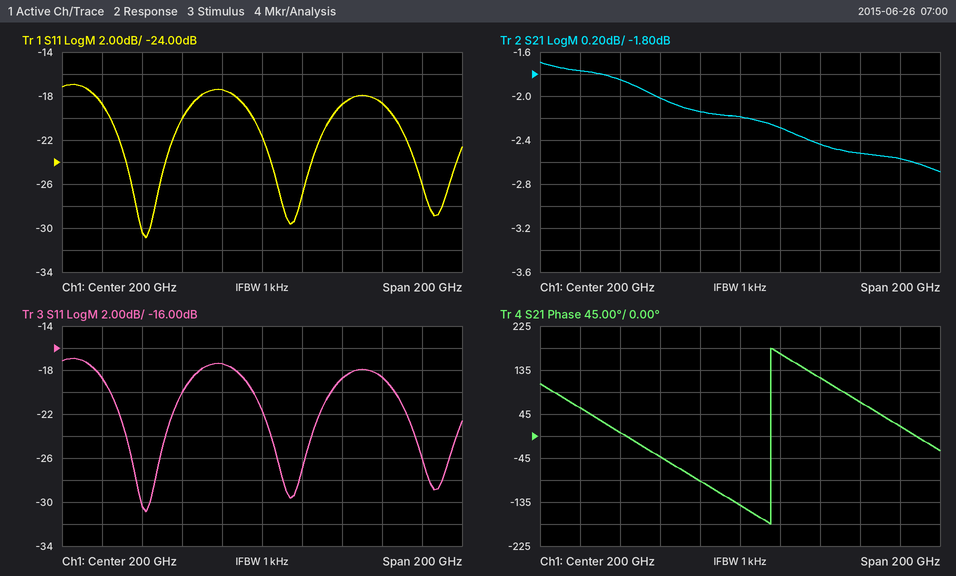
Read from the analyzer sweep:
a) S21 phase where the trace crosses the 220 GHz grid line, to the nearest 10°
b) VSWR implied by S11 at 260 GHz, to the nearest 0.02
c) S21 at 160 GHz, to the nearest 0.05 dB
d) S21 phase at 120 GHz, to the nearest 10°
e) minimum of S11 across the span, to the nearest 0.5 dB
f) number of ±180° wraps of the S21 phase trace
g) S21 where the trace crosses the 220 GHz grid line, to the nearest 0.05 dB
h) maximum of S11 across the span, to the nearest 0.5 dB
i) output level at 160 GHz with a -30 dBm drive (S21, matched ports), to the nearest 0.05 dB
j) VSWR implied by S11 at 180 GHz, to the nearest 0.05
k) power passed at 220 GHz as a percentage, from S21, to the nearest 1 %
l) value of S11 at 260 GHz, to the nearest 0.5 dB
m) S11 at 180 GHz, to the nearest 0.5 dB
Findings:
170°
1.26
-2.00 dB
60°
-31.0 dB
1
-2.30 dB
-17.0 dB
-32.00 dBm
1.30
59 %
-18.5 dB
-17.5 dB
